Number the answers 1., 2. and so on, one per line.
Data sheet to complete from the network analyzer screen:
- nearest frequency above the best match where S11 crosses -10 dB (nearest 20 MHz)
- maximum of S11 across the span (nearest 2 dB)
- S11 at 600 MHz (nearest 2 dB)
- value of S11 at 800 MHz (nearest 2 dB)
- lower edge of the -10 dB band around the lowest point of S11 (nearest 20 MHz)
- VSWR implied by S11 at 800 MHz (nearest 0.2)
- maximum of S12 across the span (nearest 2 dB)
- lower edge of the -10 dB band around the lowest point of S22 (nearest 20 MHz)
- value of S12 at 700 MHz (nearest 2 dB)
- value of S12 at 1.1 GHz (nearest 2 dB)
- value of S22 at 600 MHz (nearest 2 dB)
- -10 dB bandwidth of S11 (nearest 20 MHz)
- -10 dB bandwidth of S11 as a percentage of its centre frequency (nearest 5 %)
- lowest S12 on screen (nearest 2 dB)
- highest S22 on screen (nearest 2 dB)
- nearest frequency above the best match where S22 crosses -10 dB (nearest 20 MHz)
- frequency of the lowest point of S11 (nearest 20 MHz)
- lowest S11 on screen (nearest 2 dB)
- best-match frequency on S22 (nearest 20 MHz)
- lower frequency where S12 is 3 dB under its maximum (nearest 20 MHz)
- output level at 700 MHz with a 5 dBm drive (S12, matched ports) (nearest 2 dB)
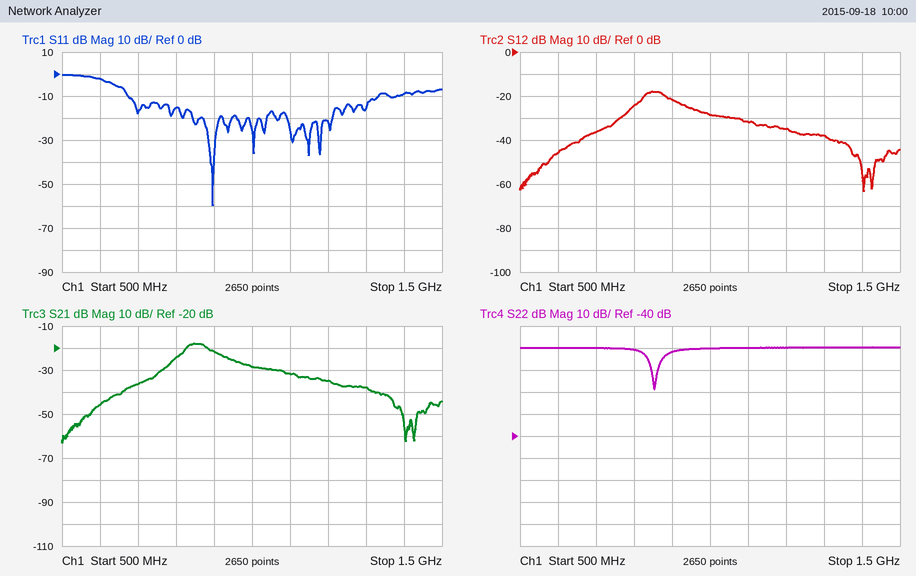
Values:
1. 1.34 GHz
2. 0 dB
3. -2 dB
4. -16 dB
5. 680 MHz
6. 1.4
7. -18 dB
8. 840 MHz
9. -36 dB
10. -32 dB
11. 0 dB
12. 660 MHz
13. 65 %
14. -64 dB
15. 0 dB
16. 860 MHz
17. 900 MHz
18. -60 dB
19. 860 MHz
20. 820 MHz
21. -32 dBm
